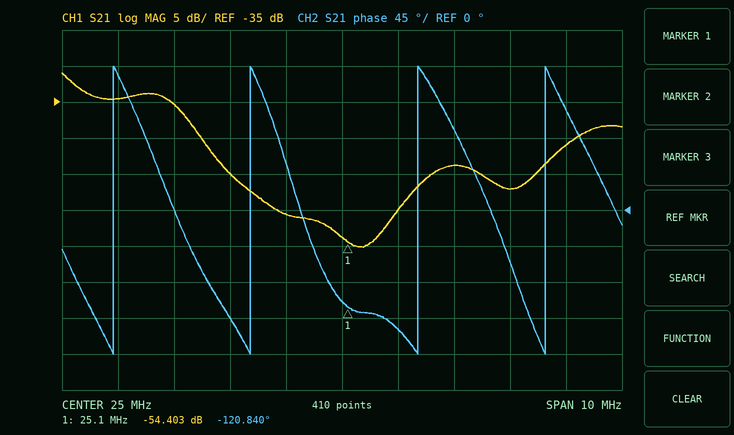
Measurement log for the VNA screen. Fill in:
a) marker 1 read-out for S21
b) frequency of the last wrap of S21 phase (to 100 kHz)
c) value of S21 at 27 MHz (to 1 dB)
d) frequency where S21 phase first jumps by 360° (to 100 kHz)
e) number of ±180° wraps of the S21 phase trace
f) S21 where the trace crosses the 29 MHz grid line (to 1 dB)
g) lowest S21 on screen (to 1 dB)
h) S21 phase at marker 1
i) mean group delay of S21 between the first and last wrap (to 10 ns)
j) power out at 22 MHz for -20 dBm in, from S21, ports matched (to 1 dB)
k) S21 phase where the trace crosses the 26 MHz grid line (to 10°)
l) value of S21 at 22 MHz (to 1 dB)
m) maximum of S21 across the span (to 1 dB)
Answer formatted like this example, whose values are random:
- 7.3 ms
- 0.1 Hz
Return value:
- -54.403 dB
- 28.6 MHz
- -44 dB
- 20.9 MHz
- 4
- -41 dB
- -55 dB
- -120.840°
- 390 ns
- -55 dBm
- -150°
- -35 dB
- -31 dB
